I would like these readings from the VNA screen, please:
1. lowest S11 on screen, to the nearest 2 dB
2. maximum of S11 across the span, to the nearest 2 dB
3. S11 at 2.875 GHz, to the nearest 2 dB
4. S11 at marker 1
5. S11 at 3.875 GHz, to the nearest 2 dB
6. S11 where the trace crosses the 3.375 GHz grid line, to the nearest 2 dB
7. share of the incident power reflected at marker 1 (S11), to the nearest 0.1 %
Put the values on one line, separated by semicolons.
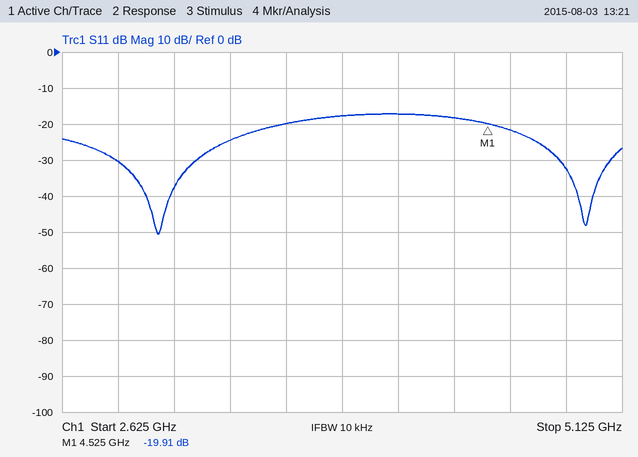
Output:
-50 dB; -18 dB; -30 dB; -19.91 dB; -18 dB; -24 dB; 1.0 %
